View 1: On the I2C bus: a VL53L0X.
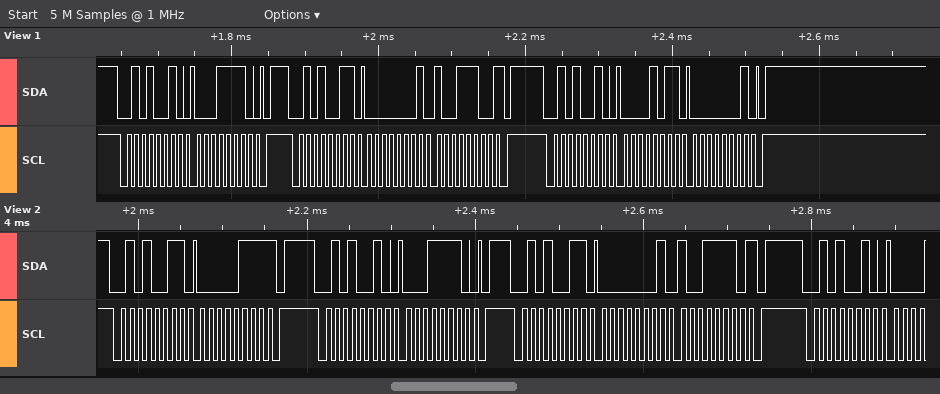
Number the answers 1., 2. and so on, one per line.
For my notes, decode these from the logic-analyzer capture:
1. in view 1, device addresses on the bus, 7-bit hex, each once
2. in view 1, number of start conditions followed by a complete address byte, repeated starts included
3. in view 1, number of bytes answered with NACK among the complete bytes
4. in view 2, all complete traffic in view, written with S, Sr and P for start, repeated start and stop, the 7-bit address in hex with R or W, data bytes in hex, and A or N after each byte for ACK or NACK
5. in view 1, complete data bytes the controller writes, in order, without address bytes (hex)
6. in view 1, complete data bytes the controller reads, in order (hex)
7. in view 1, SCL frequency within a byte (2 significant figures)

1. 0x29
2. 3
3. 1
4. S 29R A 07 N P S 29W A 1E A P S 29R A 01 A 9E N P S 29W A
5. 1E 0B 01
6. 01 9C
7. 100 kHz
